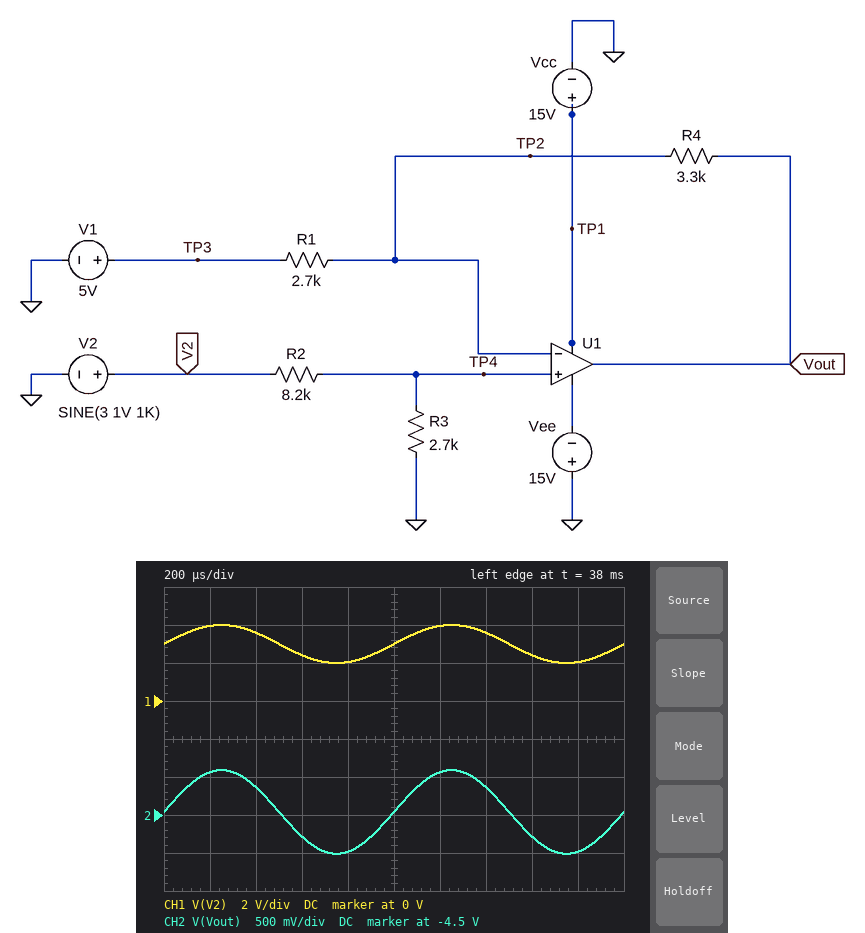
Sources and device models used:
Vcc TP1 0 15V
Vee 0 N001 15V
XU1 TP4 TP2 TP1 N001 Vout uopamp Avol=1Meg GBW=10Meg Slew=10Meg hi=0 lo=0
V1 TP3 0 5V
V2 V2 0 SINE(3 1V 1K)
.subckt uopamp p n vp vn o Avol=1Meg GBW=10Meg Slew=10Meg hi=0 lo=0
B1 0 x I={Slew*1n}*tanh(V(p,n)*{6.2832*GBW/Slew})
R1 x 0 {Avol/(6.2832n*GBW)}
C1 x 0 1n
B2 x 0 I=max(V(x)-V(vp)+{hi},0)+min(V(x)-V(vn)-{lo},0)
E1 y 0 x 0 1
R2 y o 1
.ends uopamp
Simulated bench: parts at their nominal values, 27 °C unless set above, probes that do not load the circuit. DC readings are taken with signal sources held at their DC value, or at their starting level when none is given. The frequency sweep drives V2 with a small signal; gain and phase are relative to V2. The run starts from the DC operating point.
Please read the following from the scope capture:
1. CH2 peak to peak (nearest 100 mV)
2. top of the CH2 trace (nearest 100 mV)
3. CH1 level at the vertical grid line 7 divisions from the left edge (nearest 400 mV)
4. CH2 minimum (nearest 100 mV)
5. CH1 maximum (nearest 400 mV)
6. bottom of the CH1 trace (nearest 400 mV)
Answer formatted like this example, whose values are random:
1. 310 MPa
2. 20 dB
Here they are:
1. 1.1 V
2. -3.9 V
3. 3.6 V
4. -5.0 V
5. 4.0 V
6. 2.0 V
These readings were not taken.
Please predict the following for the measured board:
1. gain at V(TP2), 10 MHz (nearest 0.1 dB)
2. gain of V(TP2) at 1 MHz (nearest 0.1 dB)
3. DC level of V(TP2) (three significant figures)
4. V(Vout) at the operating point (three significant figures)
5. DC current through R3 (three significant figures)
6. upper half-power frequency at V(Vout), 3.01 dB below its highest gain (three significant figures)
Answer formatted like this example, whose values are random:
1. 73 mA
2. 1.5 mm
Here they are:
1. -19.9 dB
2. -12.3 dB
3. 743 mV
4. -4.46 V
5. 275 µA
6. 4.50 MHz
